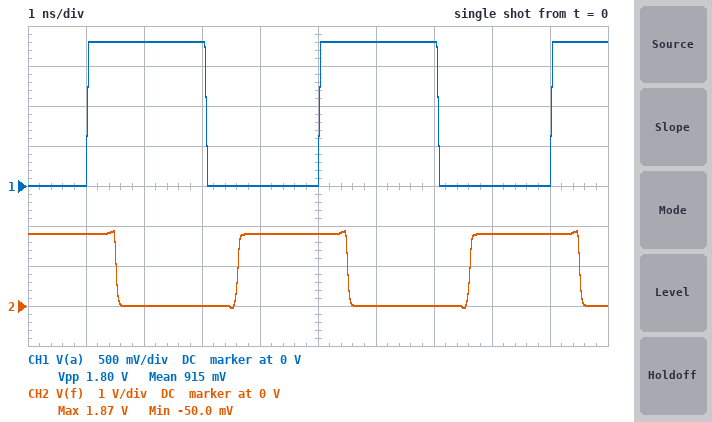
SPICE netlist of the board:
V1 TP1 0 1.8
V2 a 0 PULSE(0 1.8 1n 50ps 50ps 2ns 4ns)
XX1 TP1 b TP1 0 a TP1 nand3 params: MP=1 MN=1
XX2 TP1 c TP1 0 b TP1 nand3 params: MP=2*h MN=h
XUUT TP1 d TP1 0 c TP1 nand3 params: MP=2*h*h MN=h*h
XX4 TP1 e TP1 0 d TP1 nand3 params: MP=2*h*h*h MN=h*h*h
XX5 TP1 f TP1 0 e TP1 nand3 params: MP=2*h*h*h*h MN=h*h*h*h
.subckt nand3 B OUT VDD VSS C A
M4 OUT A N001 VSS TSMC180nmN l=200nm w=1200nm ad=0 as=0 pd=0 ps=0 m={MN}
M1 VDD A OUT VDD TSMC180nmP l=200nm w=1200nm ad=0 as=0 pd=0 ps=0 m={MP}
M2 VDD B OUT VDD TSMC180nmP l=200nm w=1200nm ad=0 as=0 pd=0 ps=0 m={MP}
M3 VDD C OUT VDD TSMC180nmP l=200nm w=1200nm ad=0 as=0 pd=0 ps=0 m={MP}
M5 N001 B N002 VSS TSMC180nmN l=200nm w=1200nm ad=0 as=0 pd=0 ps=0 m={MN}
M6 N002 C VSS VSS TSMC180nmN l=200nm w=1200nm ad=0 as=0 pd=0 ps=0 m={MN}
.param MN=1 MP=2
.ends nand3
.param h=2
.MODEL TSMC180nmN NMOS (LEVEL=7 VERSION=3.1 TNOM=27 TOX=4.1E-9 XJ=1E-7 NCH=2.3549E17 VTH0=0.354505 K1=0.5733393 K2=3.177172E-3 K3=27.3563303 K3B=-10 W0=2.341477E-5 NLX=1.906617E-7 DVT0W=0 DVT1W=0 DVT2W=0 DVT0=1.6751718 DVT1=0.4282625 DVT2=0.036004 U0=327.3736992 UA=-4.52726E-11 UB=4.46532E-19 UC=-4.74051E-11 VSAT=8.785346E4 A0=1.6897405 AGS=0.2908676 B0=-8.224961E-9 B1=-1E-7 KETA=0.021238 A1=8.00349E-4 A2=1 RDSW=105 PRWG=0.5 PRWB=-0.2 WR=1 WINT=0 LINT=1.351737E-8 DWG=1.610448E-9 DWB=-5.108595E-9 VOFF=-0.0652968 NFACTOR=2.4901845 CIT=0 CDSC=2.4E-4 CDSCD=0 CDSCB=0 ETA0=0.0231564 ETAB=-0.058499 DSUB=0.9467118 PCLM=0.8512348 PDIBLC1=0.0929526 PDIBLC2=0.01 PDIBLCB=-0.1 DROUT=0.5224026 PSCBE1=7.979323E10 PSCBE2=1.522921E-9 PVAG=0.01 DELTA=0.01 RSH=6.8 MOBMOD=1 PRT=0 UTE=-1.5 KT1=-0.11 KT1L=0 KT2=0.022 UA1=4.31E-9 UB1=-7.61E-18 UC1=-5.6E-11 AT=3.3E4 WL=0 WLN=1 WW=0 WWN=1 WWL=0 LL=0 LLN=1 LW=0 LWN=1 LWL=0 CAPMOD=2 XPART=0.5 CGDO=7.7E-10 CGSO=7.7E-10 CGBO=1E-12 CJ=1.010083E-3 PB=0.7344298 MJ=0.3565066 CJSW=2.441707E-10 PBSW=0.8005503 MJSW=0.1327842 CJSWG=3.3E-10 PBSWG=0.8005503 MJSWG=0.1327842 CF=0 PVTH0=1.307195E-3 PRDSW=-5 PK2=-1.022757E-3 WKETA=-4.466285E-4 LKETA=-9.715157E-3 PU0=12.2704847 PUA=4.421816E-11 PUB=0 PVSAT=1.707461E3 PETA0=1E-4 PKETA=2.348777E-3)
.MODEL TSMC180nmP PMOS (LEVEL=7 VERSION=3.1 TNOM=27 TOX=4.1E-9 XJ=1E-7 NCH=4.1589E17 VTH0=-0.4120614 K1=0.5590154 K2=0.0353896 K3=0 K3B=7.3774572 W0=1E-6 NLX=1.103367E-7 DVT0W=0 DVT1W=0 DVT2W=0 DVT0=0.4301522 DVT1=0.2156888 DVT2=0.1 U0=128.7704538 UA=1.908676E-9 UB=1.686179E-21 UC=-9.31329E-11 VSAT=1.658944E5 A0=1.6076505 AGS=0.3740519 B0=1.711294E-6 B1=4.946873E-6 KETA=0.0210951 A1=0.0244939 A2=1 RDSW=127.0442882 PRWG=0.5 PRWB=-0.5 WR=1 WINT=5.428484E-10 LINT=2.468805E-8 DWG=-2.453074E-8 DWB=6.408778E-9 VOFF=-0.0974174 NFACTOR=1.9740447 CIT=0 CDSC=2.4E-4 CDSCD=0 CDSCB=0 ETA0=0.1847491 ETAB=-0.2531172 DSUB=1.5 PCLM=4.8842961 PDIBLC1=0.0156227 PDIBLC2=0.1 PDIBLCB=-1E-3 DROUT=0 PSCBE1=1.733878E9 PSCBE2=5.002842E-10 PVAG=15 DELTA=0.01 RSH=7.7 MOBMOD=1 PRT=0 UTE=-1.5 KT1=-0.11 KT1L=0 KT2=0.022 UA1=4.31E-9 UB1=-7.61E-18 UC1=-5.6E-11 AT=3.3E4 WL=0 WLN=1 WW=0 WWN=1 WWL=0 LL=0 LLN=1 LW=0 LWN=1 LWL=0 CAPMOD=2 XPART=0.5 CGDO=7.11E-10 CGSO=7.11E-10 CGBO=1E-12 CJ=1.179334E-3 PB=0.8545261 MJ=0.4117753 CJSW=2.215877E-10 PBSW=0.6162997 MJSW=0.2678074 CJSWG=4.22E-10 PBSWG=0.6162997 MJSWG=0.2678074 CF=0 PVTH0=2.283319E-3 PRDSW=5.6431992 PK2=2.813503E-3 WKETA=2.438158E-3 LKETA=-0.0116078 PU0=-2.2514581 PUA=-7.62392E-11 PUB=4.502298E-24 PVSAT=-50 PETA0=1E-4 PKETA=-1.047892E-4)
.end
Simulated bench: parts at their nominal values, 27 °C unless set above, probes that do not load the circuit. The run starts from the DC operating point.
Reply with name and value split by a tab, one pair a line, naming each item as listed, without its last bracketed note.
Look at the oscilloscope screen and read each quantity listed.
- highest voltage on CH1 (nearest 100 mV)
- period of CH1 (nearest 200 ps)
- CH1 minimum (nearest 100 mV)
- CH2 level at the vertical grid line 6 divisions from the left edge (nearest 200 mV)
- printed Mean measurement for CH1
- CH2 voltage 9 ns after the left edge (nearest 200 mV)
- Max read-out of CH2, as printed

highest voltage on CH1	1.8 V
period of CH1	4.0 ns
CH1 minimum	0 V
CH2 level at the vertical grid line 6 divisions from the left edge	0 V
printed Mean measurement for CH1	915 mV
CH2 voltage 9 ns after the left edge	1.8 V
Max read-out of CH2, as printed	1.87 V
